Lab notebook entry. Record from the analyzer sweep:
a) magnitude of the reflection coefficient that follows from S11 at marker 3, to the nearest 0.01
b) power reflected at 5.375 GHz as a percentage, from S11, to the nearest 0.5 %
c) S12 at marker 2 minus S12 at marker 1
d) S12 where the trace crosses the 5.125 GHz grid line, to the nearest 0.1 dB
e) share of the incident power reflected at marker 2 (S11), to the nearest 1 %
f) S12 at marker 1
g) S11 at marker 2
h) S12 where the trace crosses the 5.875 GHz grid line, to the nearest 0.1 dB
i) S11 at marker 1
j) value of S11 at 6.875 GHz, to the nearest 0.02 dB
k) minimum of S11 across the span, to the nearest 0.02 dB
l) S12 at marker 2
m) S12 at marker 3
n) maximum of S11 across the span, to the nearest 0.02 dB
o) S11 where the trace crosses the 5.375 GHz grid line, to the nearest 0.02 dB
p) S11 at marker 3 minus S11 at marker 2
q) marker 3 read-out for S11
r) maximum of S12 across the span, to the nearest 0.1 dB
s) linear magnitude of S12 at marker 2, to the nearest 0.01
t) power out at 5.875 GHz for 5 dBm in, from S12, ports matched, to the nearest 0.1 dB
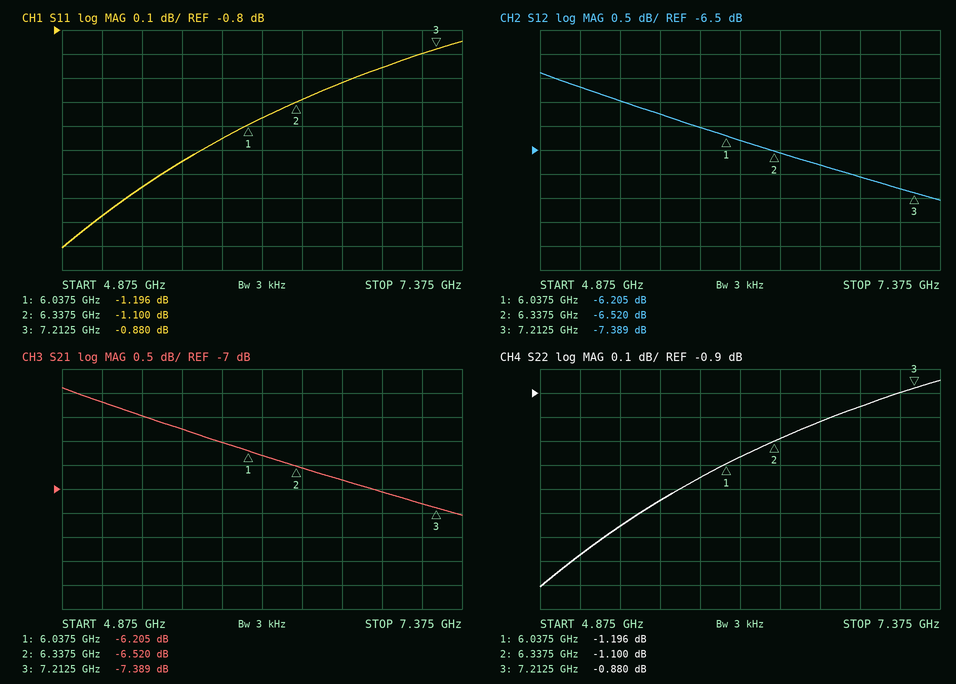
0.90
71.5 %
-0.315 dB
-5.2 dB
78 %
-6.205 dB
-1.100 dB
-6.0 dB
-1.196 dB
-0.96 dB
-1.70 dB
-6.520 dB
-7.389 dB
-0.84 dB
-1.46 dB
0.220 dB
-0.880 dB
-4.9 dB
0.47
-1.0 dBm
